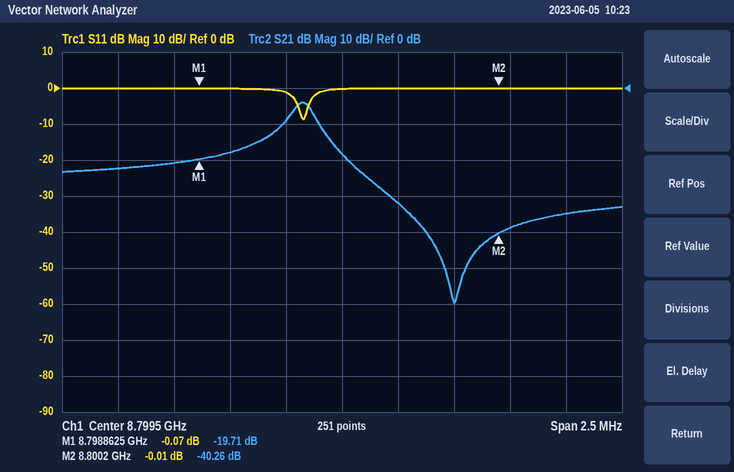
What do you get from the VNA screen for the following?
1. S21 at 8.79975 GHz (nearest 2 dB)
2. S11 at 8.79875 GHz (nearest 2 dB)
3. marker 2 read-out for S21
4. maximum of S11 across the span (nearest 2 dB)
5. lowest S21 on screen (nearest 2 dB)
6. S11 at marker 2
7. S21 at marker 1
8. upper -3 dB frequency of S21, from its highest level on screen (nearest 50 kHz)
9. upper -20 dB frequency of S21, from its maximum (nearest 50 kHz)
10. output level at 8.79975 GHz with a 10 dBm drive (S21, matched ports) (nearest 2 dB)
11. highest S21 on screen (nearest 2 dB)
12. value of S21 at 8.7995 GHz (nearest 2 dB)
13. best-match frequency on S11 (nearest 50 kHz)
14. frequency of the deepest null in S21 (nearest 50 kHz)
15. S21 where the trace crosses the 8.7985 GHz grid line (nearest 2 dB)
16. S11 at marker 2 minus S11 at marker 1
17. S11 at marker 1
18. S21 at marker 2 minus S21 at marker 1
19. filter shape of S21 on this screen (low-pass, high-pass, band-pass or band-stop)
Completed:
-32 dB
0 dB
-40.26 dB
0 dB
-60 dB
-0.01 dB
-19.71 dB
8.79935 GHz
8.79960 GHz
-22 dBm
-4 dB
-18 dB
8.79935 GHz
8.80000 GHz
-22 dB
0.06 dB
-0.07 dB
-20.55 dB
band-pass
